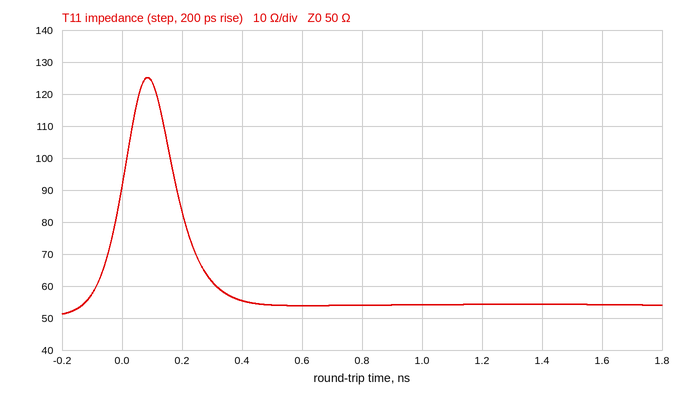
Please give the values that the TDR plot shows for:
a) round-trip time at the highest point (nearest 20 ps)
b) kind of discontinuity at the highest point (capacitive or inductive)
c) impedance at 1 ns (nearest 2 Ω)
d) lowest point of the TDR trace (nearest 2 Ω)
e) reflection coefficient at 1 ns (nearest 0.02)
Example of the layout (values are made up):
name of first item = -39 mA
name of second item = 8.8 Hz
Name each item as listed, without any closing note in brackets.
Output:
round-trip time at the highest point = 80 ps
kind of discontinuity at the highest point = inductive
impedance at 1 ns = 54 Ω
lowest point of the TDR trace = 52 Ω
reflection coefficient at 1 ns = +0.04
